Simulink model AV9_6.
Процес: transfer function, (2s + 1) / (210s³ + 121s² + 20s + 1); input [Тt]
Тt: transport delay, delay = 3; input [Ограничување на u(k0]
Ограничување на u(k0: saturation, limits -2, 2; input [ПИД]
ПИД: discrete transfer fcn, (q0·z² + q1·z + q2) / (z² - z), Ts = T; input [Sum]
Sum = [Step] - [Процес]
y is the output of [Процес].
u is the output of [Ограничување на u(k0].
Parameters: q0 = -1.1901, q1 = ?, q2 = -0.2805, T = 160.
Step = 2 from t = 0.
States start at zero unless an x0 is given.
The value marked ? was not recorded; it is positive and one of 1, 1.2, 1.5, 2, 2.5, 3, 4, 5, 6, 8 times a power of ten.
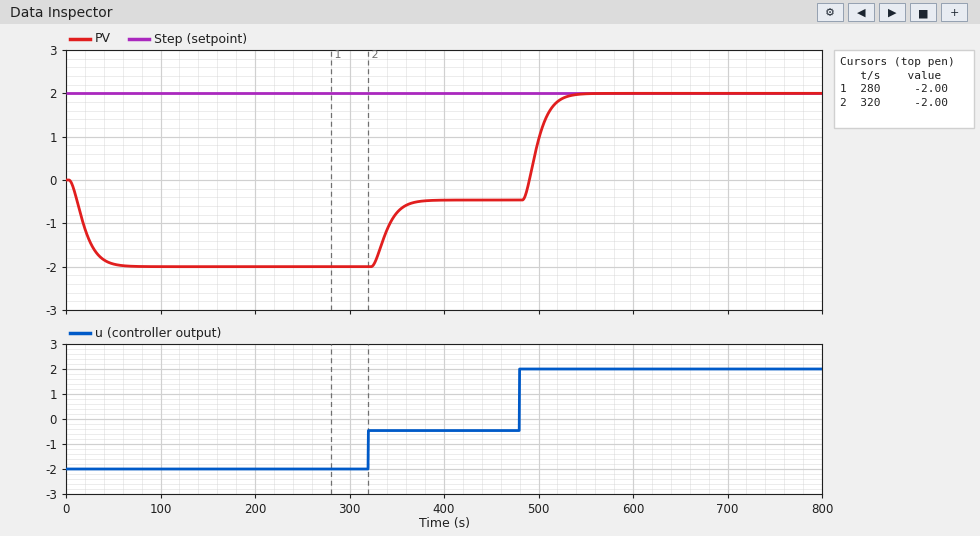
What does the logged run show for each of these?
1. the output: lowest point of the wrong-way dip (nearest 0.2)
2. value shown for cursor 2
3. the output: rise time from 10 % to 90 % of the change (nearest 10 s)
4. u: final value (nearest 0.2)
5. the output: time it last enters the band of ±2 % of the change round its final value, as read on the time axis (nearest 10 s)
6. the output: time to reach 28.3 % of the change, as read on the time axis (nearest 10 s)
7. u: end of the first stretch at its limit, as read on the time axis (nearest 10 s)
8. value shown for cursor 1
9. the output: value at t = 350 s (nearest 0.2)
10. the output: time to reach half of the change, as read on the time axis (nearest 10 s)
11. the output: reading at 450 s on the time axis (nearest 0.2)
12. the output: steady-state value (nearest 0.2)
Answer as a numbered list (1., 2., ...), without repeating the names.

1. -2.0
2. -2.00
3. 30 s
4. 2.0
5. 540 s
6. 500 s
7. 320 s
8. -2.00
9. -0.8
10. 500 s
11. -0.4
12. 2.0
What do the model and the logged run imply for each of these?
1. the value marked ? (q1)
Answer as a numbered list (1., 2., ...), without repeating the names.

1. 2
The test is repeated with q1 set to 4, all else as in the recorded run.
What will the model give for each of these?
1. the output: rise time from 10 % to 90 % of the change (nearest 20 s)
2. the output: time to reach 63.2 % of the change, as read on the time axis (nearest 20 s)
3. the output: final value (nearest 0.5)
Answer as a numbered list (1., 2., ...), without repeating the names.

1. 160 s
2. 340 s
3. 2.0
